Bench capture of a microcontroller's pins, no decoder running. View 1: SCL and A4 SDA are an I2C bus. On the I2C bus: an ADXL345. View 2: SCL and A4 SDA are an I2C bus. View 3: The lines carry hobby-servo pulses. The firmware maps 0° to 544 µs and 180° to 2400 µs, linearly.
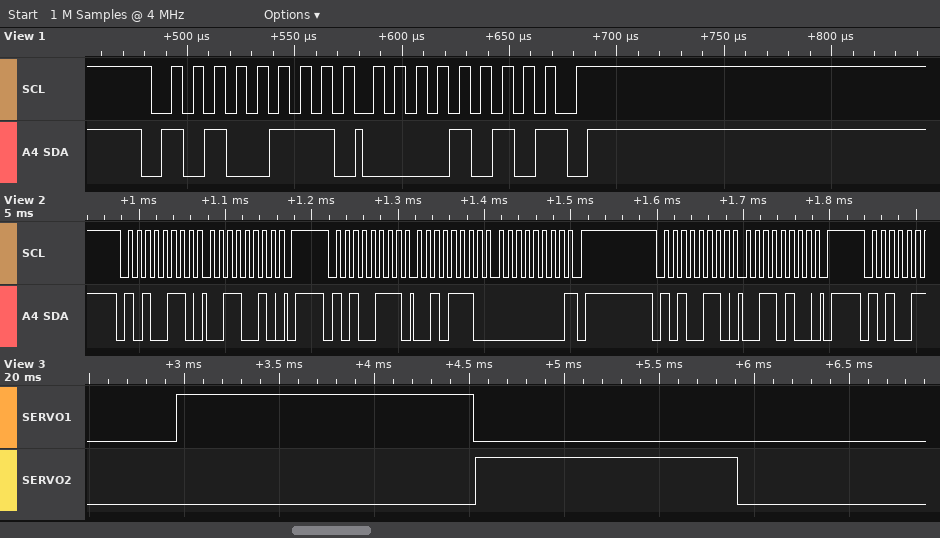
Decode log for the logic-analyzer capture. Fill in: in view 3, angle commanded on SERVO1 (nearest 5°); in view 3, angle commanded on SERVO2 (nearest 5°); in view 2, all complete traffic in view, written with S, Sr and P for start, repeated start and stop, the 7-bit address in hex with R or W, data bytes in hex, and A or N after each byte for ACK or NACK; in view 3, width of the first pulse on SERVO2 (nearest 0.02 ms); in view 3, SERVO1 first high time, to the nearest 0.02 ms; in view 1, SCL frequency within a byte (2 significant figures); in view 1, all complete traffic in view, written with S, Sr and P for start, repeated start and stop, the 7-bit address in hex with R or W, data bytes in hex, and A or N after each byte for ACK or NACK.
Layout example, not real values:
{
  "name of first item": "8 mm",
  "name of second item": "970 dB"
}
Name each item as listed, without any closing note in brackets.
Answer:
{
  "in view 3, angle commanded on SERVO1": "100°",
  "in view 3, angle commanded on SERVO2": "80°",
  "in view 2, all complete traffic in view, written with S, Sr and P for start, repeated start and stop, the 7-bit address in hex with R or W, data bytes in hex, and A or N after each byte for ACK or NACK": "S 53W A 32 A P S 53R A 2E A 00 N P S 53W A 34 A P",
  "in view 3, width of the first pulse on SERVO2": "1.38 ms",
  "in view 3, SERVO1 first high time, to the nearest 0.02 ms": "1.56 ms",
  "in view 1, SCL frequency within a byte": "100 kHz",
  "in view 1, all complete traffic in view, written with S, Sr and P for start, repeated start and stop, the 7-bit address in hex with R or W, data bytes in hex, and A or N after each byte for ACK or NACK": "S 53R A 0A N P"
}
